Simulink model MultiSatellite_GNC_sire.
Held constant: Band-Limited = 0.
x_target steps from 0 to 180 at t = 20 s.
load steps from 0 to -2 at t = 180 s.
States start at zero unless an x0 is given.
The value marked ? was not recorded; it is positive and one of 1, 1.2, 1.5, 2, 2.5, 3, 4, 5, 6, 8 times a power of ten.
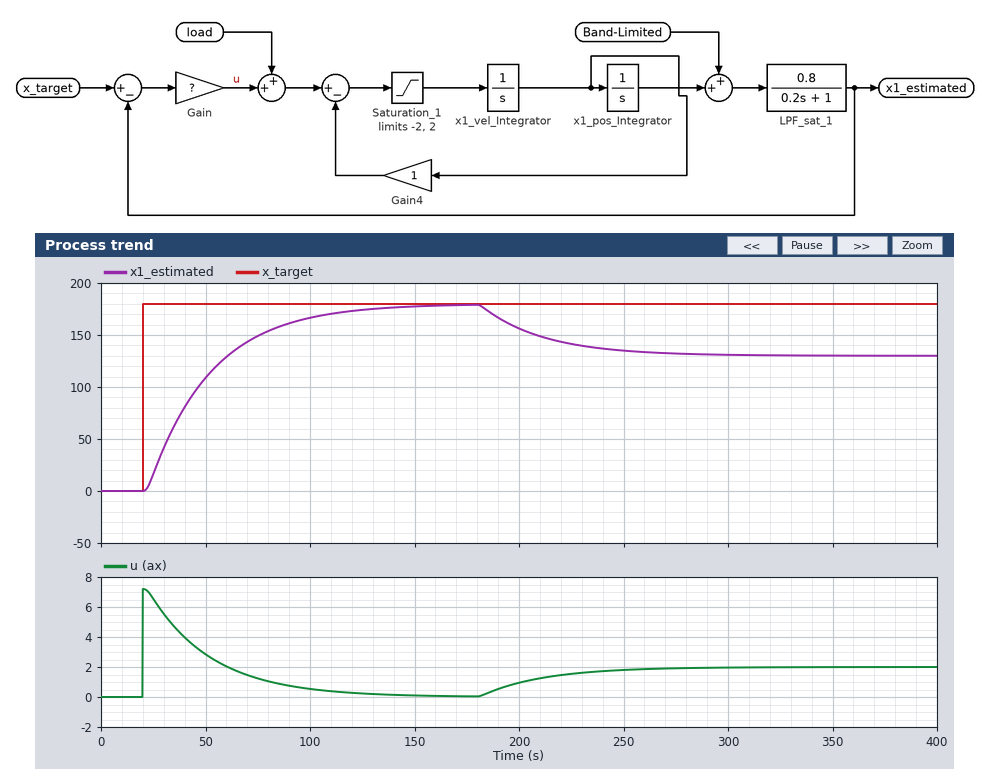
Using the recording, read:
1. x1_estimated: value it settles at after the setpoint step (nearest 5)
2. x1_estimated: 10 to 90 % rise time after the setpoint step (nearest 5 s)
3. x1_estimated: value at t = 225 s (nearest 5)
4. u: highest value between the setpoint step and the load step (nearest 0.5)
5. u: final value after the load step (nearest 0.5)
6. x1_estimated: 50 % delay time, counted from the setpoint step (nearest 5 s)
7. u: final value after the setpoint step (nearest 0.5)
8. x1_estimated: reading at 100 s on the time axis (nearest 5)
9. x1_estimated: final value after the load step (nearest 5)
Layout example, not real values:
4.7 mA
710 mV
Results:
180
65 s
140
7.0
2.0
25 s
0.0
165
130
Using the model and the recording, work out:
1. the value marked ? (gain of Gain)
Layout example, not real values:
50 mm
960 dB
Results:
0.04
